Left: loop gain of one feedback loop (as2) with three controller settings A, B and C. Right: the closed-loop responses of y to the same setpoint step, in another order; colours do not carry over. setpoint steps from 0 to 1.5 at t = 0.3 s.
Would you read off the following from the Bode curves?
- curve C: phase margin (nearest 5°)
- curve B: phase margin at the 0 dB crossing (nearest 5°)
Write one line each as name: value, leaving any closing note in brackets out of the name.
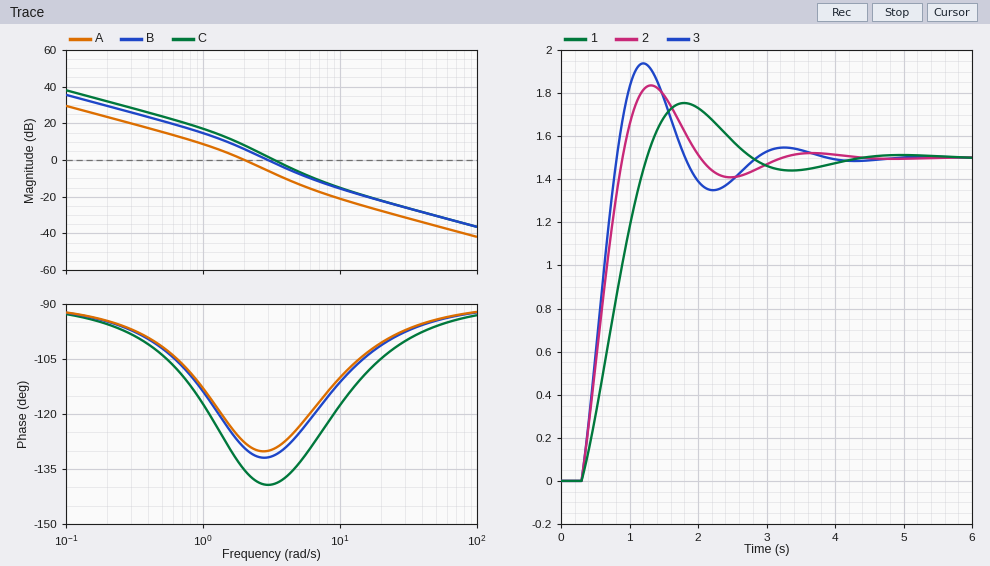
curve C: phase margin: 40°
curve B: phase margin at the 0 dB crossing: 50°
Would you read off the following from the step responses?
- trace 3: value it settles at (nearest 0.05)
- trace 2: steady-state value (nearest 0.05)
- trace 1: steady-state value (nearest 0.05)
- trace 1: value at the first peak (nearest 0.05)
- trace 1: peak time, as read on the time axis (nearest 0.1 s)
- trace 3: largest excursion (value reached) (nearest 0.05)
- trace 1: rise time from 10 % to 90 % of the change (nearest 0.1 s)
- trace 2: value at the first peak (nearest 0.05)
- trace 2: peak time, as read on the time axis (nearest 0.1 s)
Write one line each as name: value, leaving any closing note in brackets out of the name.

trace 3: value it settles at: 1.50
trace 2: steady-state value: 1.50
trace 1: steady-state value: 1.50
trace 1: value at the first peak: 1.75
trace 1: peak time, as read on the time axis: 1.8 s
trace 3: largest excursion (value reached): 1.95
trace 1: rise time from 10 % to 90 % of the change: 0.7 s
trace 2: value at the first peak: 1.85
trace 2: peak time, as read on the time axis: 1.3 s
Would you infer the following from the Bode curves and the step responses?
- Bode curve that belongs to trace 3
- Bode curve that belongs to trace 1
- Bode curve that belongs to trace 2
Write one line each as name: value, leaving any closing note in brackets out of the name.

Bode curve that belongs to trace 3: C
Bode curve that belongs to trace 1: A
Bode curve that belongs to trace 2: B
